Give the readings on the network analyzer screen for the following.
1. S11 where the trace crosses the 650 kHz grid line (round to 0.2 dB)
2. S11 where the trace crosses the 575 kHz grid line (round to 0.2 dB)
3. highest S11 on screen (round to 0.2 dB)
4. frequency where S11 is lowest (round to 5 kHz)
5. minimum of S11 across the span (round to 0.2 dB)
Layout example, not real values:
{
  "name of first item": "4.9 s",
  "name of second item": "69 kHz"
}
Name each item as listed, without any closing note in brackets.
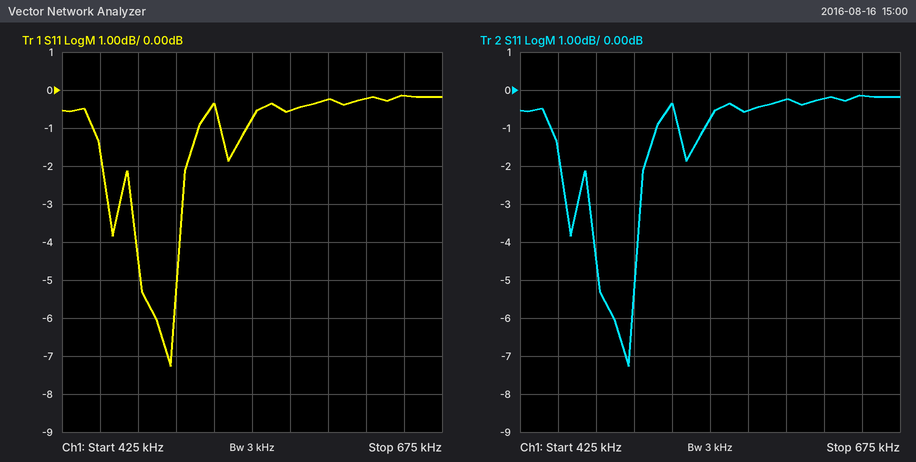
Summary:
{
  "S11 where the trace crosses the 650 kHz grid line": "-0.2 dB",
  "S11 where the trace crosses the 575 kHz grid line": "-0.6 dB",
  "highest S11 on screen": "-0.2 dB",
  "frequency where S11 is lowest": "495 kHz",
  "minimum of S11 across the span": "-7.2 dB"
}
